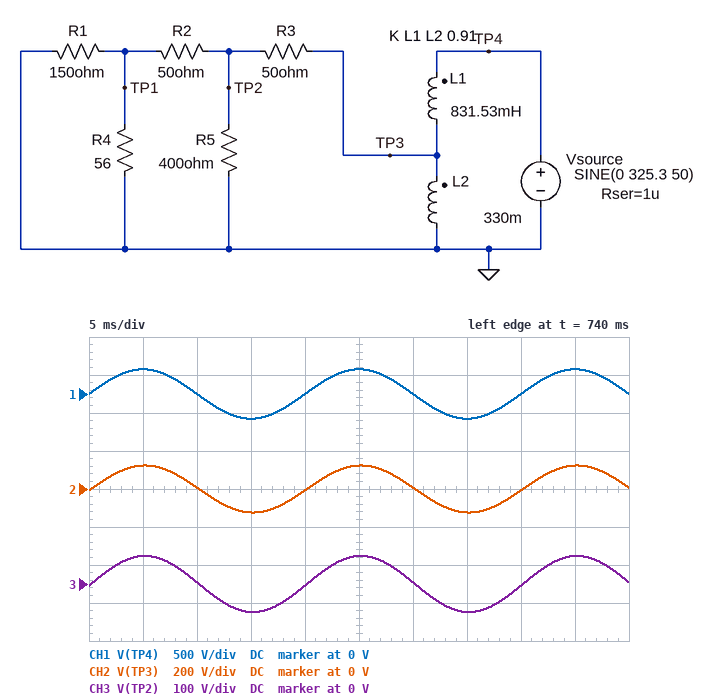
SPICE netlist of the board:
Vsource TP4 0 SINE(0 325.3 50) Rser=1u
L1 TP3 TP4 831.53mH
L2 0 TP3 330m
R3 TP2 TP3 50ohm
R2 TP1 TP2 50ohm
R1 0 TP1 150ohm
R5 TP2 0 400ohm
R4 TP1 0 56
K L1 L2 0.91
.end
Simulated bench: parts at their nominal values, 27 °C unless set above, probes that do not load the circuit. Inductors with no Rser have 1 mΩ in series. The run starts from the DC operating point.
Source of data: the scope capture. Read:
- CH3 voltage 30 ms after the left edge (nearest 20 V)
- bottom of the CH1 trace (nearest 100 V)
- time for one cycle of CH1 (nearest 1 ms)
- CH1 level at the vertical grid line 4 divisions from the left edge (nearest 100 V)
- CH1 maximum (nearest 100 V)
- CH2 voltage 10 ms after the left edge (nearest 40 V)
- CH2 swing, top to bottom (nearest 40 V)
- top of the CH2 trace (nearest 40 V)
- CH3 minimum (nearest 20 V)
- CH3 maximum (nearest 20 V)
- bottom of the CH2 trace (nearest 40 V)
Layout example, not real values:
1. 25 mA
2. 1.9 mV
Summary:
1. 0 V
2. -300 V
3. 20 ms
4. 0 V
5. 300 V
6. 0 V
7. 240 V
8. 120 V
9. -80 V
10. 80 V
11. -120 V
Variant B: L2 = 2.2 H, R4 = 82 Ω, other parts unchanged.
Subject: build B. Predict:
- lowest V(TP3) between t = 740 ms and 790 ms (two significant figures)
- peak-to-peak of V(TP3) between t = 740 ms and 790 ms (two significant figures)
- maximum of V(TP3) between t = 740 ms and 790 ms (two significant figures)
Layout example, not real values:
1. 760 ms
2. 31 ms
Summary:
1. -200 V
2. 400 V
3. 200 V
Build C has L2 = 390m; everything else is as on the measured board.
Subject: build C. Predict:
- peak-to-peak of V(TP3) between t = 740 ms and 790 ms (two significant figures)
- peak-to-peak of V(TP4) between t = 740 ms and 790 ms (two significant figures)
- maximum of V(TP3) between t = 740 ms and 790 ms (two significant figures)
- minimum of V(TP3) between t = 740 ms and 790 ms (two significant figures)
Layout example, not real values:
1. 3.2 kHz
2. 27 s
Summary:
1. 260 V
2. 650 V
3. 130 V
4. -130 V
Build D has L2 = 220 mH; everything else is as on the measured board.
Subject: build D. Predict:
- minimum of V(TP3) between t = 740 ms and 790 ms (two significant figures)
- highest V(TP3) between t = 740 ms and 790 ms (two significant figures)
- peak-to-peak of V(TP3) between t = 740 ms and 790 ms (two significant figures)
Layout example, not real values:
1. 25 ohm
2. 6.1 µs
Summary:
1. -110 V
2. 110 V
3. 220 V
